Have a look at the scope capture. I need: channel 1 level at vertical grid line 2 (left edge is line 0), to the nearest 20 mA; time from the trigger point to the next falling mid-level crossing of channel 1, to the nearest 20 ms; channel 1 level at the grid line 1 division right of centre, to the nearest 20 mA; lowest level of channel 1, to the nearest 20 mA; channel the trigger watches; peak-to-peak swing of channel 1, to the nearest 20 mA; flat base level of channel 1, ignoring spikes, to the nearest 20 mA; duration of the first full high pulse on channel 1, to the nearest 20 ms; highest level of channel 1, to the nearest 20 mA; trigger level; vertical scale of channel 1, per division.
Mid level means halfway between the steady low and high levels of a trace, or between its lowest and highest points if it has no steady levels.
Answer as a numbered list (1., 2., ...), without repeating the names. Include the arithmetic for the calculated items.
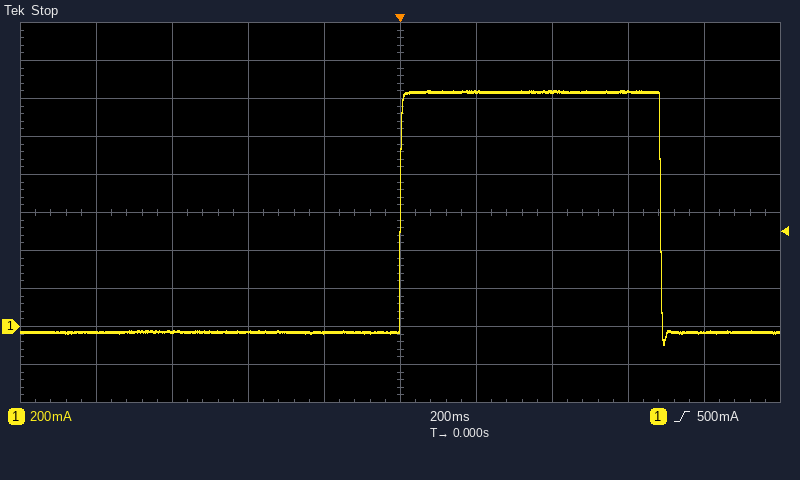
1. -20 mA
2. 680 ms
3. 1.24 A
4. -100 mA
5. channel 1
6. 1.24 A − (-100 mA) = 1.34 A
7. -20 mA
8. 680 ms
9. 1.24 A
10. 500 mA
11. 200 mA
